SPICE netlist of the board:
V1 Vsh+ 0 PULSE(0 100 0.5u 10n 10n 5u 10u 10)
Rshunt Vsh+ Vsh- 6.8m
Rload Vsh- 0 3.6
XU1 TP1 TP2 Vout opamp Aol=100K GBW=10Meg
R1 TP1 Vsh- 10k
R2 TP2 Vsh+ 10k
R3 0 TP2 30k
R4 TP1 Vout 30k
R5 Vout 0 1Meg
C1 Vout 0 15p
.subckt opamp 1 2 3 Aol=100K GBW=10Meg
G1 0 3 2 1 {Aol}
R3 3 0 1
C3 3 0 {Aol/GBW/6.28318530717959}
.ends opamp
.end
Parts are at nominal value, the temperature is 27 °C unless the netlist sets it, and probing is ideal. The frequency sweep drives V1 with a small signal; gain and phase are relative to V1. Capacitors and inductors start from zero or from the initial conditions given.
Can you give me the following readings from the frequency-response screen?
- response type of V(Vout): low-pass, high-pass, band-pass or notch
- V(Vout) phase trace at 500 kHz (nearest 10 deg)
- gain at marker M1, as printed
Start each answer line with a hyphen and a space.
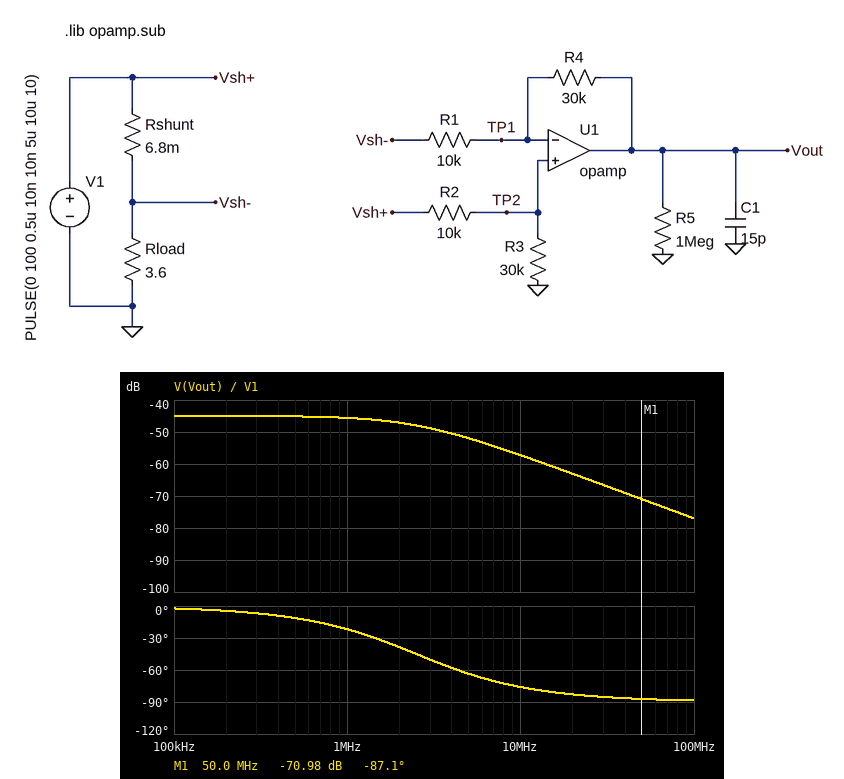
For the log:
- low-pass
- -10 deg
- -70.98 dB
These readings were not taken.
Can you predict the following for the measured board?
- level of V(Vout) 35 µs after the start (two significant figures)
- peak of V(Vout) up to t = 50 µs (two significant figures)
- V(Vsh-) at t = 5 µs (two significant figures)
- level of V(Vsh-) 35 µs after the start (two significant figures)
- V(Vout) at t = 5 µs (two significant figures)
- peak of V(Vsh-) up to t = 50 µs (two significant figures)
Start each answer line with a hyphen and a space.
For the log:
- 570 mV
- 570 mV
- 100 V
- 100 V
- 570 mV
- 100 V
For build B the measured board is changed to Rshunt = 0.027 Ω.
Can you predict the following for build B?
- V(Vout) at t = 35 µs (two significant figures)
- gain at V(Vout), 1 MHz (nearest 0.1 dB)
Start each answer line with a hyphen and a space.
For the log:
- 2.2 V
- -33.7 dB
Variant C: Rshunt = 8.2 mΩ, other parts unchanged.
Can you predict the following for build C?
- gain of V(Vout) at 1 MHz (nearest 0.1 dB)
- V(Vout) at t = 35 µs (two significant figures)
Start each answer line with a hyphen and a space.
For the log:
- -44.0 dB
- 680 mV
